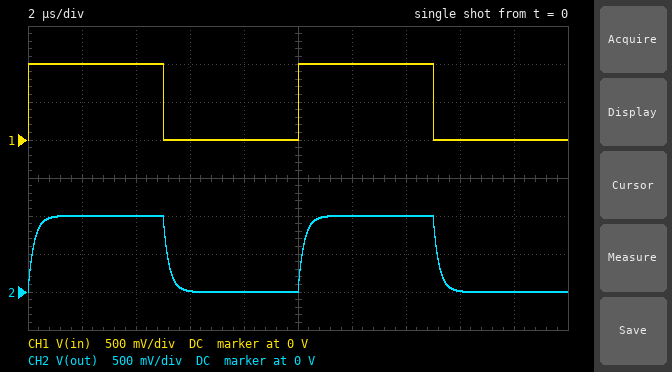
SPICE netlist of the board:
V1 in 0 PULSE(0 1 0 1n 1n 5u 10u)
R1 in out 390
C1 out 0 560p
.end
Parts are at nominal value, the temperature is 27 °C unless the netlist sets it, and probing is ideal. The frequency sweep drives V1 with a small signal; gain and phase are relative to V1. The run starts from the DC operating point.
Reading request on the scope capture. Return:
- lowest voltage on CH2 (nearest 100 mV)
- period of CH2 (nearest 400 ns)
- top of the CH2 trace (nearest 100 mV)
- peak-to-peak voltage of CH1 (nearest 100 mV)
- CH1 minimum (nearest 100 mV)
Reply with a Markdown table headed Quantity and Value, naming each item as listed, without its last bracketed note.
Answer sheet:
| Quantity | Value |
|---|---|
| lowest voltage on CH2 | 0 V |
| period of CH2 | 10.0 µs |
| top of the CH2 trace | 1.0 V |
| peak-to-peak voltage of CH1 | 1.0 V |
| CH1 minimum | 0 V |
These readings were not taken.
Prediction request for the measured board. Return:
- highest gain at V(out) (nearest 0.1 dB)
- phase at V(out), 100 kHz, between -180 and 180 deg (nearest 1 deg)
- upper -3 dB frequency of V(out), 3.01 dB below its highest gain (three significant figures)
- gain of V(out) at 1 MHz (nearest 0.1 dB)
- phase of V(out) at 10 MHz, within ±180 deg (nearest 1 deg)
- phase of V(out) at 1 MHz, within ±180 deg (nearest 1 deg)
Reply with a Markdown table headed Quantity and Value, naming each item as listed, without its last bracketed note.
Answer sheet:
| Quantity | Value |
|---|---|
| highest gain at V(out) | 0 dB |
| phase at V(out), 100 kHz, between -180 and 180 deg | -8 deg |
| upper -3 dB frequency of V(out), 3.01 dB below its highest gain | 729 kHz |
| gain of V(out) at 1 MHz | -4.6 dB |
| phase of V(out) at 10 MHz, within ±180 deg | -86 deg |
| phase of V(out) at 1 MHz, within ±180 deg | -54 deg |
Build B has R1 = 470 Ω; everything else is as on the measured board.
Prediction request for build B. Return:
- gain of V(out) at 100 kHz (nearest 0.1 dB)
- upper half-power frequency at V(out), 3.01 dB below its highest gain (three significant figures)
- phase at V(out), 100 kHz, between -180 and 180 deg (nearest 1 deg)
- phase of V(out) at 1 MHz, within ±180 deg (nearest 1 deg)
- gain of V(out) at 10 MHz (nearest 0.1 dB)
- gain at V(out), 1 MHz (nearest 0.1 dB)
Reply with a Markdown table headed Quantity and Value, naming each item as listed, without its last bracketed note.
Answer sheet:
| Quantity | Value |
|---|---|
| gain of V(out) at 100 kHz | -0.1 dB |
| upper half-power frequency at V(out), 3.01 dB below its highest gain | 605 kHz |
| phase at V(out), 100 kHz, between -180 and 180 deg | -9 deg |
| phase of V(out) at 1 MHz, within ±180 deg | -59 deg |
| gain of V(out) at 10 MHz | -24.4 dB |
| gain at V(out), 1 MHz | -5.7 dB |
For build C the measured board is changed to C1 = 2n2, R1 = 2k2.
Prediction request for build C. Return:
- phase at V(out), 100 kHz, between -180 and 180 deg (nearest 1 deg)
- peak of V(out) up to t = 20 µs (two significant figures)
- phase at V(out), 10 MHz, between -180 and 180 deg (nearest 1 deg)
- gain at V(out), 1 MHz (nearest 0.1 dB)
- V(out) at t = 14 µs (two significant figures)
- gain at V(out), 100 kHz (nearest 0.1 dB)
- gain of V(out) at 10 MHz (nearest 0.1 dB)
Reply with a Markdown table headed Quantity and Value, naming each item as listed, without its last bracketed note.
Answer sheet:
| Quantity | Value |
|---|---|
| phase at V(out), 100 kHz, between -180 and 180 deg | -72 deg |
| peak of V(out) up to t = 20 µs | 730 mV |
| phase at V(out), 10 MHz, between -180 and 180 deg | -90 deg |
| gain at V(out), 1 MHz | -29.7 dB |
| V(out) at t = 14 µs | 660 mV |
| gain at V(out), 100 kHz | -10.1 dB |
| gain of V(out) at 10 MHz | -49.7 dB |
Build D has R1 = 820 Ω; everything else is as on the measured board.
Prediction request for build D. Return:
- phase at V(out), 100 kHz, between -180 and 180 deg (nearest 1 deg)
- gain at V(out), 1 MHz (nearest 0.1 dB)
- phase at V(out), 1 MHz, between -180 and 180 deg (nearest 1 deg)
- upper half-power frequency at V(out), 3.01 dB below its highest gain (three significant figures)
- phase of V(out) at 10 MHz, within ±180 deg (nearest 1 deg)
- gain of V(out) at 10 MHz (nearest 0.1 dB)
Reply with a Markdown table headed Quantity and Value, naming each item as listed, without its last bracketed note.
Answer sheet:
| Quantity | Value |
|---|---|
| phase at V(out), 100 kHz, between -180 and 180 deg | -16 deg |
| gain at V(out), 1 MHz | -9.7 dB |
| phase at V(out), 1 MHz, between -180 and 180 deg | -71 deg |
| upper half-power frequency at V(out), 3.01 dB below its highest gain | 347 kHz |
| phase of V(out) at 10 MHz, within ±180 deg | -88 deg |
| gain of V(out) at 10 MHz | -29.2 dB |
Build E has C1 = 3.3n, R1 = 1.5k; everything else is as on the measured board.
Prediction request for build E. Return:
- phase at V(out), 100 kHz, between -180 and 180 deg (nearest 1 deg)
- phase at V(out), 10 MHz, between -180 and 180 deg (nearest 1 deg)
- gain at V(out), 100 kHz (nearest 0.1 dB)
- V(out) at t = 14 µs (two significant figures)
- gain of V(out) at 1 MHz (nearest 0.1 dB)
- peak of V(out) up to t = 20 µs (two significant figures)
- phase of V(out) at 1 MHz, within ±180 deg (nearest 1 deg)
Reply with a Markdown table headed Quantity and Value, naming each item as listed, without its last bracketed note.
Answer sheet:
| Quantity | Value |
|---|---|
| phase at V(out), 100 kHz, between -180 and 180 deg | -72 deg |
| phase at V(out), 10 MHz, between -180 and 180 deg | -90 deg |
| gain at V(out), 100 kHz | -10.3 dB |
| V(out) at t = 14 µs | 660 mV |
| gain of V(out) at 1 MHz | -29.9 dB |
| peak of V(out) up to t = 20 µs | 720 mV |
| phase of V(out) at 1 MHz, within ±180 deg | -88 deg |
